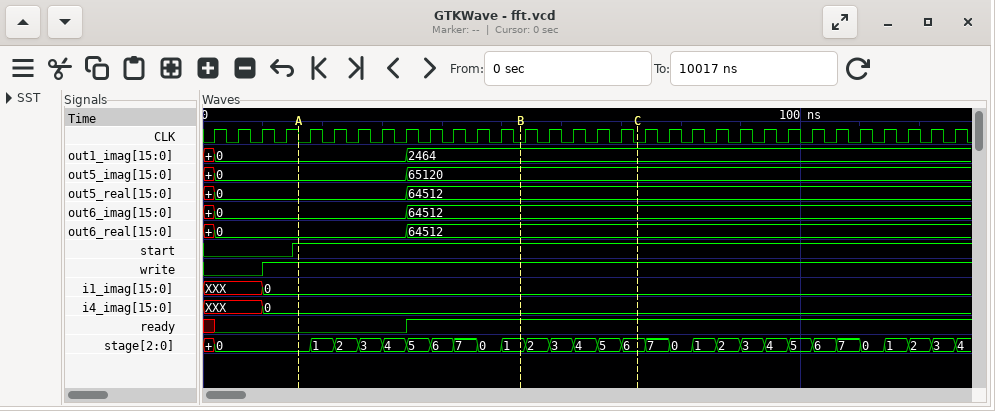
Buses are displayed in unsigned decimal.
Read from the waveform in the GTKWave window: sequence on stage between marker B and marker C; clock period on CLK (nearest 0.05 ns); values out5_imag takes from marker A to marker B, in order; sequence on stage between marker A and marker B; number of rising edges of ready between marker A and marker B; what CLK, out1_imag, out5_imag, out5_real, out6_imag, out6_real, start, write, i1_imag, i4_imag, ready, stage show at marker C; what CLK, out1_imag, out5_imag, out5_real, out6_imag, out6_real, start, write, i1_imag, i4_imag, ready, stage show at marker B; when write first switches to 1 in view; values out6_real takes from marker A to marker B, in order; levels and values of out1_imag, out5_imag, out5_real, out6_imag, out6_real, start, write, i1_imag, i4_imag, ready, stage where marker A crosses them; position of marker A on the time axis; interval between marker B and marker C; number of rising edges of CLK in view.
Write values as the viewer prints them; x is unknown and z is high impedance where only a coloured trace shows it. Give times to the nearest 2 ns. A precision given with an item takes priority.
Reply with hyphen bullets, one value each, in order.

- 1, 2, 3, 4, 5, 6
- 4 ns
- 0, 65120
- 0, 1, 2, 3, 4, 5, 6, 7, 0, 1
- 1
- CLK=0, out1_imag=2464, out5_imag=65120, out5_real=64512, out6_imag=64512, out6_real=64512, start=1, write=1, i1_imag=0, i4_imag=0, ready=1, stage=6
- CLK=0, out1_imag=2464, out5_imag=65120, out5_real=64512, out6_imag=64512, out6_real=64512, start=1, write=1, i1_imag=0, i4_imag=0, ready=1, stage=1
- 10 ns
- 0, 64512
- out1_imag=0, out5_imag=0, out5_real=0, out6_imag=0, out6_real=0, start=1, write=1, i1_imag=0, i4_imag=0, ready=0, stage=0
- 16 ns
- 20 ns
- 32
